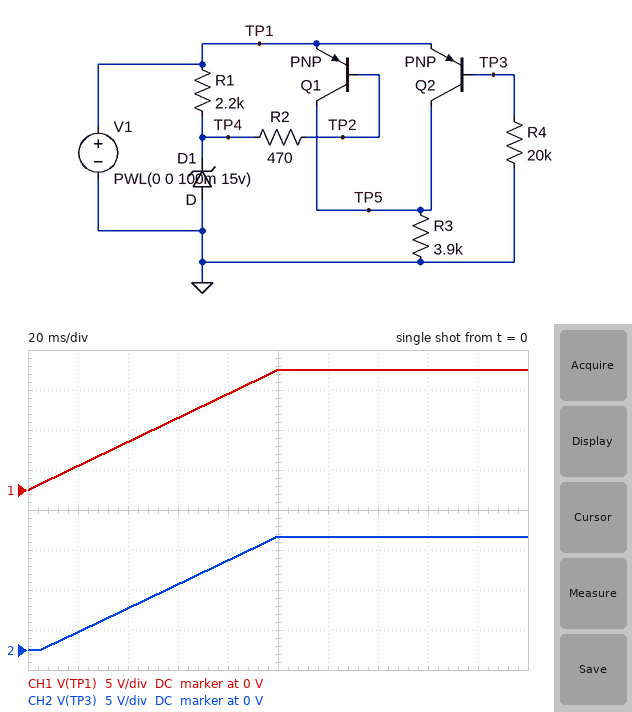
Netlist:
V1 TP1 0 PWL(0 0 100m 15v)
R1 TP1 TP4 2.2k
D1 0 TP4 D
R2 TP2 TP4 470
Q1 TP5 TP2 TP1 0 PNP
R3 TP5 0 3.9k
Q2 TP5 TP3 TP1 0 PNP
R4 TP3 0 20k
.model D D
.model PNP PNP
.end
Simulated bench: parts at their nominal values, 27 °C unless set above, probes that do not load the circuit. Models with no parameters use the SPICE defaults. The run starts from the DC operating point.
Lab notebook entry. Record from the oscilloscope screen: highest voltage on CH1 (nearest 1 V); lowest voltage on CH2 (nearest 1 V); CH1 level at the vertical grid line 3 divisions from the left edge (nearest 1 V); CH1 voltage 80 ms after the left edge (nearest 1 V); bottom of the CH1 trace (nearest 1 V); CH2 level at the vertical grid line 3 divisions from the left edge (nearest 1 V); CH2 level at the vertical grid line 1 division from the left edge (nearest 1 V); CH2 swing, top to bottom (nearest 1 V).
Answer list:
15 V
0 V
9 V
12 V
0 V
8 V
2 V
14 V
